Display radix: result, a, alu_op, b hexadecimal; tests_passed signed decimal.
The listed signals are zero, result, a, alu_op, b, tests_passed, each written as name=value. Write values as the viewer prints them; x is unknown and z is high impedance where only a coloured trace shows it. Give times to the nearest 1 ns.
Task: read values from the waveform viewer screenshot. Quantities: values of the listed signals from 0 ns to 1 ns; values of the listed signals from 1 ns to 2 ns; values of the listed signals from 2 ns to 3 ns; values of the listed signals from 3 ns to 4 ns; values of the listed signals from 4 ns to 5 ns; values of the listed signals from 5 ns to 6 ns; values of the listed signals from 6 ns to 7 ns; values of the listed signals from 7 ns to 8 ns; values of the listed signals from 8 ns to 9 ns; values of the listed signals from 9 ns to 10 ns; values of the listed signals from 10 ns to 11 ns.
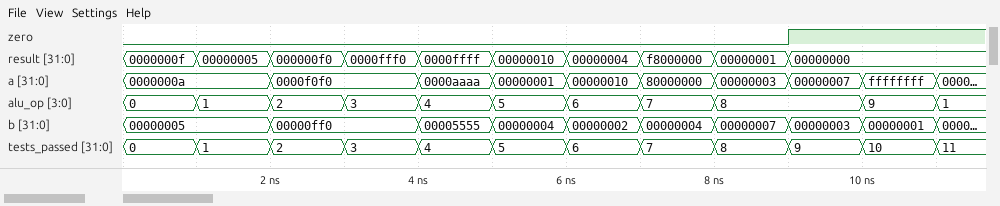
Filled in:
zero=0, result=0000000f, a=0000000a, alu_op=0, b=00000005, tests_passed=0
zero=0, result=00000005, a=0000000a, alu_op=1, b=00000005, tests_passed=1
zero=0, result=000000f0, a=0000f0f0, alu_op=2, b=00000ff0, tests_passed=2
zero=0, result=0000fff0, a=0000f0f0, alu_op=3, b=00000ff0, tests_passed=3
zero=0, result=0000ffff, a=0000aaaa, alu_op=4, b=00005555, tests_passed=4
zero=0, result=00000010, a=00000001, alu_op=5, b=00000004, tests_passed=5
zero=0, result=00000004, a=00000010, alu_op=6, b=00000002, tests_passed=6
zero=0, result=f8000000, a=80000000, alu_op=7, b=00000004, tests_passed=7
zero=0, result=00000001, a=00000003, alu_op=8, b=00000007, tests_passed=8
zero=1, result=00000000, a=00000007, alu_op=8, b=00000003, tests_passed=9
zero=1, result=00000000, a=ffffffff, alu_op=9, b=00000001, tests_passed=10
